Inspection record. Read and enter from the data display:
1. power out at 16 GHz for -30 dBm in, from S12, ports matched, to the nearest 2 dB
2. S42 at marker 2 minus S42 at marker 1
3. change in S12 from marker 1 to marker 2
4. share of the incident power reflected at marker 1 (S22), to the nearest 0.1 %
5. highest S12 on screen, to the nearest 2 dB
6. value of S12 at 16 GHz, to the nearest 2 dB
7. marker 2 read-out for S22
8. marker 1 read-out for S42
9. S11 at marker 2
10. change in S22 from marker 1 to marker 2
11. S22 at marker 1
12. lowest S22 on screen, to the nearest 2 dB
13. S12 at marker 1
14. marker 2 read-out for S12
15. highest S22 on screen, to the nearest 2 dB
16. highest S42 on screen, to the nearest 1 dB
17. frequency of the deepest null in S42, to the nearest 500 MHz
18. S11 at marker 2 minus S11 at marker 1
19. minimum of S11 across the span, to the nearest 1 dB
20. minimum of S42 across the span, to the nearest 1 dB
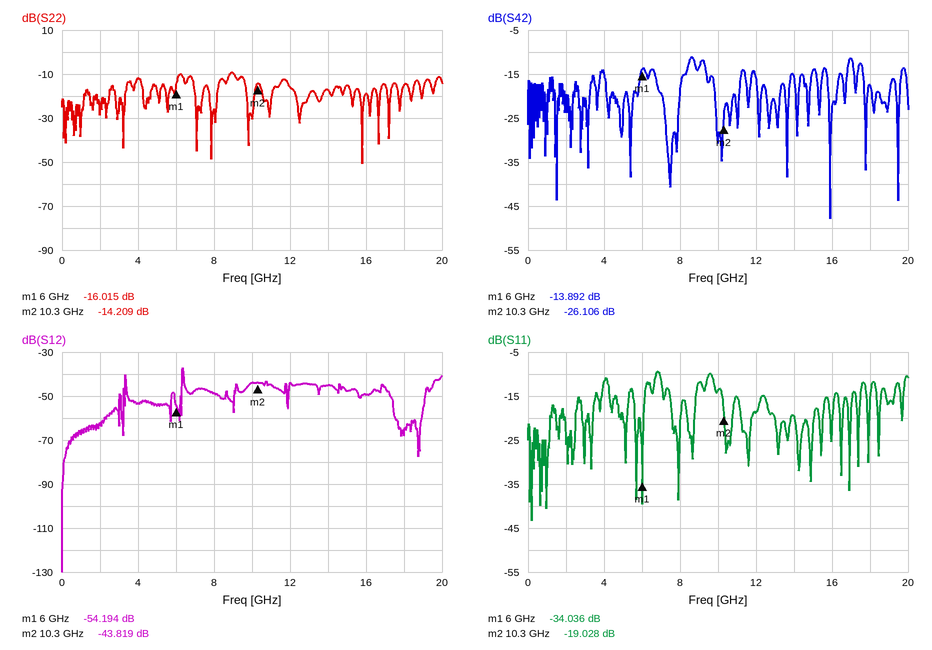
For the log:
-80 dBm
-12.214 dB
10.375 dB
2.5 %
-38 dB
-50 dB
-14.209 dB
-13.892 dB
-19.028 dB
1.806 dB
-16.015 dB
-50 dB
-54.194 dB
-43.819 dB
-10 dB
-11 dB
16.0 GHz
15.008 dB
-43 dB
-48 dB
